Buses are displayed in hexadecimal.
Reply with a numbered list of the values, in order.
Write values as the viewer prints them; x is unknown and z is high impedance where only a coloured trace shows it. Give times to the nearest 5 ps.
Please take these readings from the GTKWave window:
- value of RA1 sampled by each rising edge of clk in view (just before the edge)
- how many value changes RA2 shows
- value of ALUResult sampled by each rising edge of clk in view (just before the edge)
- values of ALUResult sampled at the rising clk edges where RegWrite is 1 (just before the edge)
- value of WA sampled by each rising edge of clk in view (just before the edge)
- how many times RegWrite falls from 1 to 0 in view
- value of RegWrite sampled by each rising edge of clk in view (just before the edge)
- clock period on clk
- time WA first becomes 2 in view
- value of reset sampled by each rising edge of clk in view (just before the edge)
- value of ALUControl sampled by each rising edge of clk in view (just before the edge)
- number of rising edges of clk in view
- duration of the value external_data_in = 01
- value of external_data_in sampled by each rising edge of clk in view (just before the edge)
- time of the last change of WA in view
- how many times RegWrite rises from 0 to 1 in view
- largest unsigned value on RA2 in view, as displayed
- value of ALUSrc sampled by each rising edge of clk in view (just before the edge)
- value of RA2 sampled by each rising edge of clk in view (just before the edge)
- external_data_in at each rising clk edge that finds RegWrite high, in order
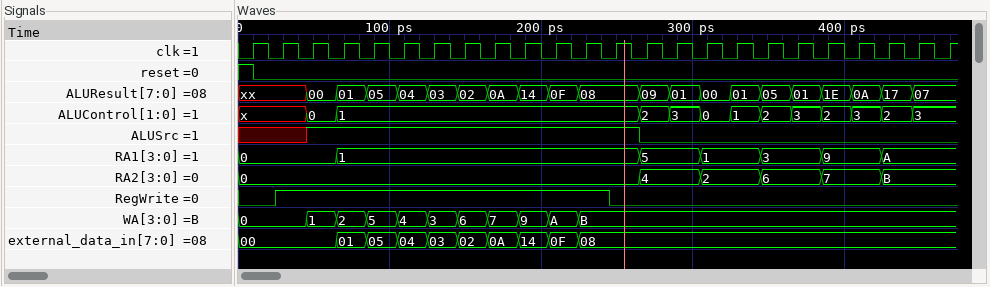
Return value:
1. 0, 0, 0, 1, 1, 1, 1, 1, 1, 1, 1, 1, 1, 5, 5, 1, 1, 3, 3, 9, 9, A, A, A
2. 5
3. xx, xx, 00, 01, 05, 04, 03, 02, 0A, 14, 0F, 08, 08, 09, 01, 00, 01, 05, 01, 1E, 0A, 17, 07, 07
4. xx, 00, 01, 05, 04, 03, 02, 0A, 14, 0F, 08
5. 0, 0, 1, 2, 5, 4, 3, 6, 7, 9, A, B, B, B, B, B, B, B, B, B, B, B, B, B
6. 1
7. 0 1 1 1 1 1 1 1 1 1 1 1 0 0 0 0 0 0 0 0 0 0 0 0
8. 20 ps
9. 65 ps
10. 1 0 0 0 0 0 0 0 0 0 0 0 0 0 0 0 0 0 0 0 0 0 0 0
11. x, x, 0, 1, 1, 1, 1, 1, 1, 1, 1, 1, 1, 2, 3, 0, 1, 2, 3, 2, 3, 2, 3, 3
12. 24
13. 20 ps
14. 00, 00, 00, 01, 05, 04, 03, 02, 0A, 14, 0F, 08, 08, 08, 08, 08, 08, 08, 08, 08, 08, 08, 08, 08
15. 225 ps
16. 1
17. B
18. x x 1 1 1 1 1 1 1 1 1 1 1 0 0 0 0 0 0 0 0 0 0 0
19. 0, 0, 0, 0, 0, 0, 0, 0, 0, 0, 0, 0, 0, 4, 4, 2, 2, 6, 6, 7, 7, B, B, B
20. 00, 00, 01, 05, 04, 03, 02, 0A, 14, 0F, 08
